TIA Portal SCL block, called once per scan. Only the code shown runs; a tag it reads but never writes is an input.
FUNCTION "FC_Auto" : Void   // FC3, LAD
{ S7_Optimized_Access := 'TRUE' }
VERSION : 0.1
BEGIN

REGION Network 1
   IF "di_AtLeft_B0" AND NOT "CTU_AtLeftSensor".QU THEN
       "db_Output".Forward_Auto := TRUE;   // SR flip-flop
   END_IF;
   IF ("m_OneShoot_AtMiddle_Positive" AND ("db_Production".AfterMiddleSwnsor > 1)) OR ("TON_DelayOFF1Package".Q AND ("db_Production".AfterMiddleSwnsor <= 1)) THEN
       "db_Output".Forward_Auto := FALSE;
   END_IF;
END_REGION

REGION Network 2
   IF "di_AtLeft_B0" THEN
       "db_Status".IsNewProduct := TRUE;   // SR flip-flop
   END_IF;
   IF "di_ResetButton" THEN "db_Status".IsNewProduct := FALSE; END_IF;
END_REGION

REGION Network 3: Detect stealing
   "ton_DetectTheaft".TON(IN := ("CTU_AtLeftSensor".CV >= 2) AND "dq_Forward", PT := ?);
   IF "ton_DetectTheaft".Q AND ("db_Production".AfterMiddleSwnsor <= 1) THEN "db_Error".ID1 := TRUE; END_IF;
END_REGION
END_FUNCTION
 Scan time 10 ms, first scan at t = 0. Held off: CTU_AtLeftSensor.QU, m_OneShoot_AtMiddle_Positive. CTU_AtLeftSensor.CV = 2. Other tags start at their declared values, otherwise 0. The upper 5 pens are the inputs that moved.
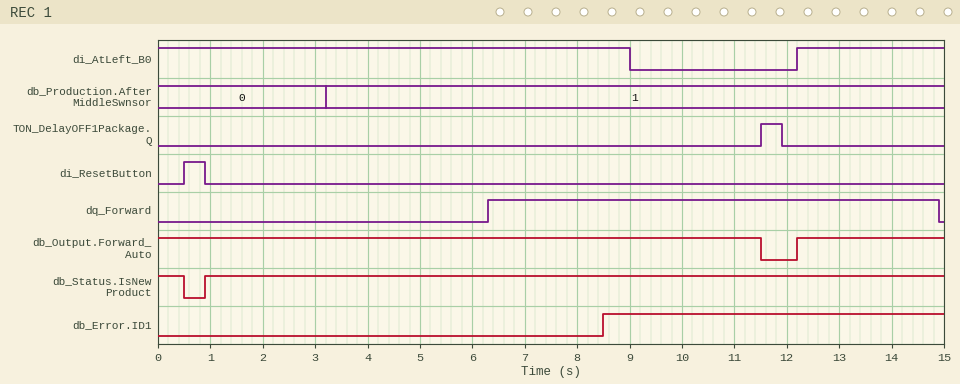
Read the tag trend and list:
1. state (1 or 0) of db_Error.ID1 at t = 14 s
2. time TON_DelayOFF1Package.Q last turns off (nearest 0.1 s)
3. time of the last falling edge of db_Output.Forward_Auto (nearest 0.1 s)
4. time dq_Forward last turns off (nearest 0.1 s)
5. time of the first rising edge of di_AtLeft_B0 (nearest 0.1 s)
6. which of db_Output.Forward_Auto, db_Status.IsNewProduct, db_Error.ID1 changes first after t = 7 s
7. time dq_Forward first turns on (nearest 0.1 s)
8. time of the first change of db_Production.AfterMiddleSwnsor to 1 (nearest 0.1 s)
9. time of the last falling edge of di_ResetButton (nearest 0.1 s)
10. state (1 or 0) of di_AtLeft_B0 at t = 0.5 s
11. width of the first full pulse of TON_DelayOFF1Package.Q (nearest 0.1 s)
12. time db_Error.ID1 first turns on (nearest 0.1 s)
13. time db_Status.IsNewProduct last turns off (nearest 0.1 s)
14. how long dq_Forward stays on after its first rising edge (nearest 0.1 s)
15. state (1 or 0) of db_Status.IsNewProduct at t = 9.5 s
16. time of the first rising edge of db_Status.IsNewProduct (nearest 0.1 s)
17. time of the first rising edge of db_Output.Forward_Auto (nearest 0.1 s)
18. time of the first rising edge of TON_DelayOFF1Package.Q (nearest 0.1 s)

1
11.9 s
11.5 s
14.9 s
12.2 s
db_Error.ID1
6.3 s
3.2 s
0.9 s
1
0.4 s
8.5 s
0.5 s
8.6 s
1
0.9 s
12.2 s
11.5 s
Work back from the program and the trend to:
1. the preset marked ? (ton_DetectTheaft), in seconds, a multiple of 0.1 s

2.2 s
